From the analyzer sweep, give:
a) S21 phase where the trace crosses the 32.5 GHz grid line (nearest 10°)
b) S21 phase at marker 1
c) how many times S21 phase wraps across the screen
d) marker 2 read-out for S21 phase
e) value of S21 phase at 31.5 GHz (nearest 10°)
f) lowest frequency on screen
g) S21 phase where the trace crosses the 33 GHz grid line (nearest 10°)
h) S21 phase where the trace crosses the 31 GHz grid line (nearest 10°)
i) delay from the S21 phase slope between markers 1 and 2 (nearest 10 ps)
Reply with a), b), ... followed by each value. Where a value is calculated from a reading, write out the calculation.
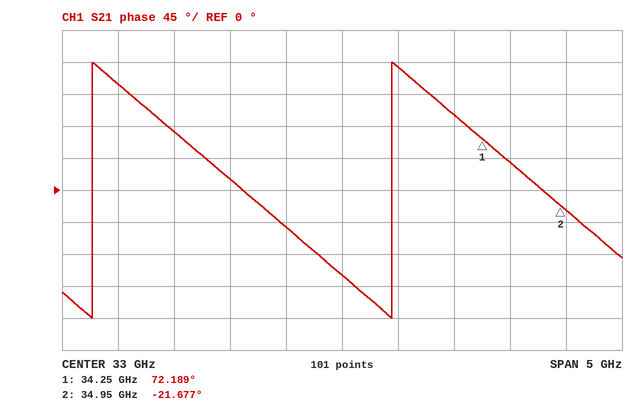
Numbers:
a) -50°
b) 72.189°
c) 2
d) -21.677°
e) 80°
f) 30.5 GHz
g) -120°
h) 150°
i) −(-21.677° − (72.189°))/(360° × 700 MHz) ≈ 372 ps, so 370 ps to the nearest 10 ps
